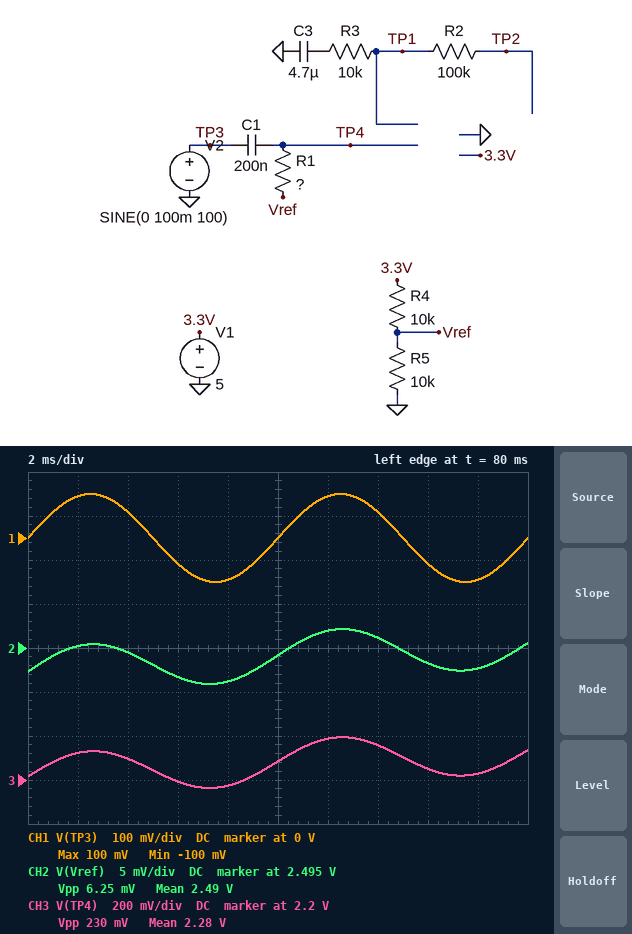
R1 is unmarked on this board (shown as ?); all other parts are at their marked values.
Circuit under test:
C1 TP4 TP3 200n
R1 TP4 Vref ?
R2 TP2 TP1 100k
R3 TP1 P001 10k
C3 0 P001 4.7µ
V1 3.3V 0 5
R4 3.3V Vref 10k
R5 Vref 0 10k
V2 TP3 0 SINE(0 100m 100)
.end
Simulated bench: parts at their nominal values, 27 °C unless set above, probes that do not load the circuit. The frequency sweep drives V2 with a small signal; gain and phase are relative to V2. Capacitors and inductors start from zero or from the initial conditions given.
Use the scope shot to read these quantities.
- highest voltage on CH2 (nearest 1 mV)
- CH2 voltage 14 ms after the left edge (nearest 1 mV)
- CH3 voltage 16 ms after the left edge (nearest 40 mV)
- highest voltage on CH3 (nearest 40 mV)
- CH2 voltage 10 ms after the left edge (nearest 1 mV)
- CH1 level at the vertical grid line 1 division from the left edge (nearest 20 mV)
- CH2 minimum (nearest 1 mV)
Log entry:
2.497 V
2.496 V
2.24 V
2.40 V
2.494 V
100 mV
2.491 V
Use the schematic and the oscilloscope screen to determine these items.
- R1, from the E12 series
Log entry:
180 kΩ
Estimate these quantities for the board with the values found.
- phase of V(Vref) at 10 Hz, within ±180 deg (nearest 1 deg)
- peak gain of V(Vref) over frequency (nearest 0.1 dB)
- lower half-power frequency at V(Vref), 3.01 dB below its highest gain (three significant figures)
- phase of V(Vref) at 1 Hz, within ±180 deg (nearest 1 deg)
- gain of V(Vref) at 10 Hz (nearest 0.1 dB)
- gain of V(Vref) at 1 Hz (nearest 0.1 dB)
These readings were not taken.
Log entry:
23 deg
-31.4 dB
4.30 Hz
77 deg
-32.1 dB
-44.3 dB
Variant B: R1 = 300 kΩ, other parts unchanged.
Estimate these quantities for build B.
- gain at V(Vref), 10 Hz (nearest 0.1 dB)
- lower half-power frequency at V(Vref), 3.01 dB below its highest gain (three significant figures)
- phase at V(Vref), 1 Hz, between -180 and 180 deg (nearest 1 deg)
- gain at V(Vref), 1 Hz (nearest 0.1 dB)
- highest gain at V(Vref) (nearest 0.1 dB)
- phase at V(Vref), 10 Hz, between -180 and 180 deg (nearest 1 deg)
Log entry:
-36.0 dB
2.61 Hz
69 deg
-44.6 dB
-35.7 dB
15 deg
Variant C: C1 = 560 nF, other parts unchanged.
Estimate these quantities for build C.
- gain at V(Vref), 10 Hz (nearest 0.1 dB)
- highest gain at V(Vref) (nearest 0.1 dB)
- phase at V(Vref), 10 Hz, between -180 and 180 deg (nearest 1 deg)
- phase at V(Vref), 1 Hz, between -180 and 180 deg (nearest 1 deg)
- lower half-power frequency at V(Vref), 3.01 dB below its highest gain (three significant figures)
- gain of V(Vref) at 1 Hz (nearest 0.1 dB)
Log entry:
-31.5 dB
-31.4 dB
9 deg
57 deg
1.54 Hz
-36.6 dB
